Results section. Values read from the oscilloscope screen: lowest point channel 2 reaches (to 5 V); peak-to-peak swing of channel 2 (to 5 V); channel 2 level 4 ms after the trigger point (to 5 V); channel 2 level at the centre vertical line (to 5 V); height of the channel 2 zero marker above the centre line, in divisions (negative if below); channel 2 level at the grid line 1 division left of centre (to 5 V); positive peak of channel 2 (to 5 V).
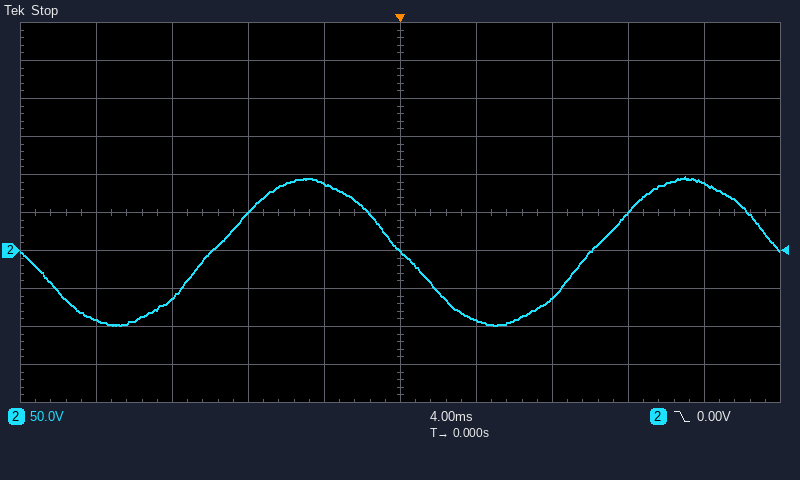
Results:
-100 V
195 V
-90 V
0 V
-1.0 div
90 V
95 V
